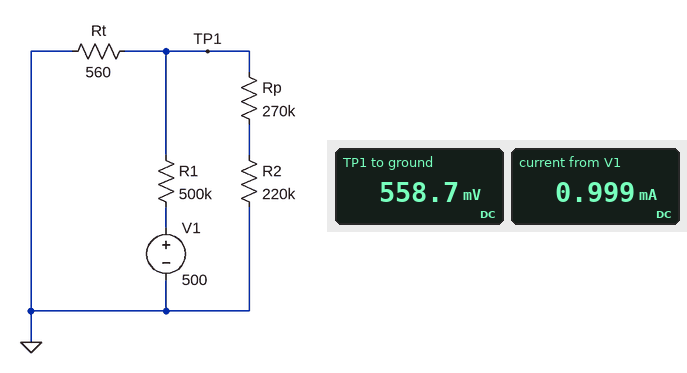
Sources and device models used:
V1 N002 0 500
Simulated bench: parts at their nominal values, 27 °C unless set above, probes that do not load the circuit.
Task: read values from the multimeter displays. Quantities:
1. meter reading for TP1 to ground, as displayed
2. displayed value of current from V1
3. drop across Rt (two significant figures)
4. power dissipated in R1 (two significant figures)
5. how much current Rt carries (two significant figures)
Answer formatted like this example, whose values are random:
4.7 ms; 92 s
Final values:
558.7 mV; 0.999 mA; 560 mV; 500 mW; 1.0 mA
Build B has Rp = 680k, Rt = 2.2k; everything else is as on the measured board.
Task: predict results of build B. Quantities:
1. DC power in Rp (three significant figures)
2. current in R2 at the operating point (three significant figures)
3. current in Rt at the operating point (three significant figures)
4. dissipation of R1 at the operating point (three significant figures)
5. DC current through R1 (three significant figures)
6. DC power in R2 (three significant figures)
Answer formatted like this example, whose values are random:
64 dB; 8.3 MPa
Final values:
4.01 µW; 2.43 µA; 993 µA; 496 mW; 996 µA; 1.30 µW
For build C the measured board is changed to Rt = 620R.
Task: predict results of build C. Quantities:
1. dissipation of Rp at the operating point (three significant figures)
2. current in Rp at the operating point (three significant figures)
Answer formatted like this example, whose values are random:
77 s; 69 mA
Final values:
430 nW; 1.26 µA
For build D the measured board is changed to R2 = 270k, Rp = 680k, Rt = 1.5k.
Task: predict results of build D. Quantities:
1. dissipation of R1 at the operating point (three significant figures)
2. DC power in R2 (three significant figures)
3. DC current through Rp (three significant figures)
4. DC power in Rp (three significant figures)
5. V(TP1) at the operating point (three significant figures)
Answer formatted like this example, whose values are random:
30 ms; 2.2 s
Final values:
497 mW; 667 nW; 1.57 µA; 1.68 µW; 1.49 V
